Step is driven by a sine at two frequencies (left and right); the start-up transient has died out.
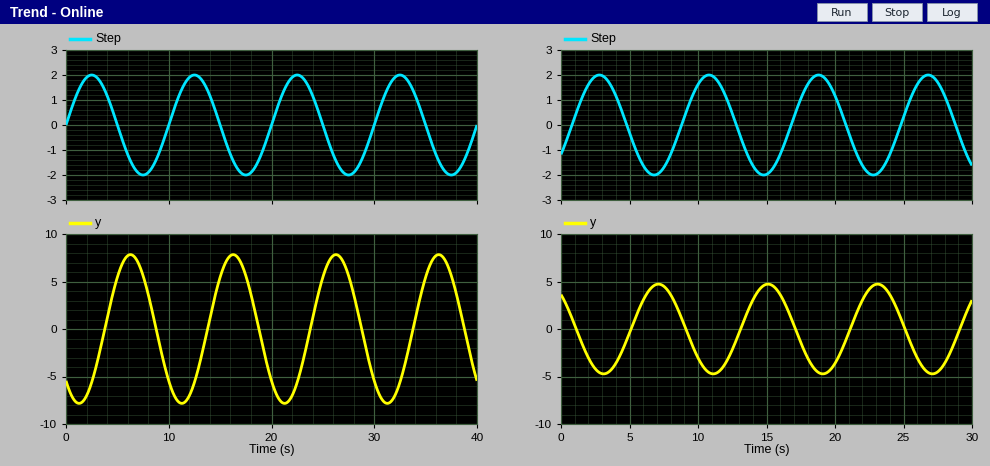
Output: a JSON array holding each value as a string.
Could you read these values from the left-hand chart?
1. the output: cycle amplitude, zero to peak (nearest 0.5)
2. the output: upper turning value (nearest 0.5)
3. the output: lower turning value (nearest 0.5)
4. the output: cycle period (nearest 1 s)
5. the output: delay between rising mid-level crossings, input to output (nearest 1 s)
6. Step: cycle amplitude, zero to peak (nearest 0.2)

["8.0", "8.0", "-8.0", "10 s", "4 s", "2.0"]
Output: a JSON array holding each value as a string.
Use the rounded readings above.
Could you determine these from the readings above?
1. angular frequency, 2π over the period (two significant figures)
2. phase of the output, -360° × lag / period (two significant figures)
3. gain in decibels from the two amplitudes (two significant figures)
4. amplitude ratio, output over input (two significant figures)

["0.63 rad/s", "-140°", "12 dB", "4.0"]
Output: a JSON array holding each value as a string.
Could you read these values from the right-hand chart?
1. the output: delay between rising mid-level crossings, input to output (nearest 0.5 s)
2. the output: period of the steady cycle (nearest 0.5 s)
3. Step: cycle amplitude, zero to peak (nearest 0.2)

["4.5 s", "8.0 s", "2.0"]
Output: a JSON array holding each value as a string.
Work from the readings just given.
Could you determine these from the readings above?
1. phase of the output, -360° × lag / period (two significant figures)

["-200°"]
